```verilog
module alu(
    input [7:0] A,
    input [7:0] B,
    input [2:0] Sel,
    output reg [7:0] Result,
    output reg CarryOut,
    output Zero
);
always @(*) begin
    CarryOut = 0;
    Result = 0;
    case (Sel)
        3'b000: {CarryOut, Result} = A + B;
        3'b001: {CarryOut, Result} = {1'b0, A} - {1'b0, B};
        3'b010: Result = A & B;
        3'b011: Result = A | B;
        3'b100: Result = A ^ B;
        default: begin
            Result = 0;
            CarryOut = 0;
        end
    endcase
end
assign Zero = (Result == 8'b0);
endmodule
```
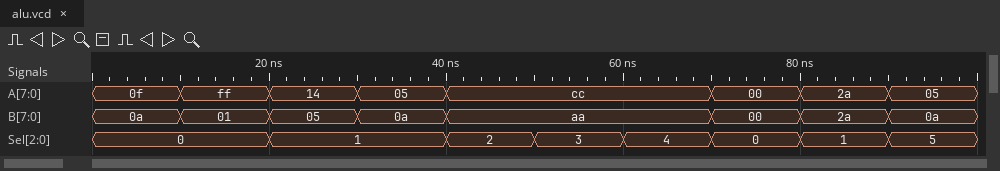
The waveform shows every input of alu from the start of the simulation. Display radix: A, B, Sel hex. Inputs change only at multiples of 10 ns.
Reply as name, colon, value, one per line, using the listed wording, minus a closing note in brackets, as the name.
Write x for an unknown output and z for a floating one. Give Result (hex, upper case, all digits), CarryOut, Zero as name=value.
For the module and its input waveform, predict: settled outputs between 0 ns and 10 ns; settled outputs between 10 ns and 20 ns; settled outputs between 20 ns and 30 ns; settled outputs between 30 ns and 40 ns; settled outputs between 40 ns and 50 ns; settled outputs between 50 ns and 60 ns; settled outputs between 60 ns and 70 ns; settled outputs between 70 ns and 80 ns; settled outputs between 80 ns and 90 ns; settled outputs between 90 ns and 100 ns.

settled outputs between 0 ns and 10 ns: Result=19, CarryOut=0, Zero=0
settled outputs between 10 ns and 20 ns: Result=00, CarryOut=1, Zero=1
settled outputs between 20 ns and 30 ns: Result=0F, CarryOut=0, Zero=0
settled outputs between 30 ns and 40 ns: Result=FB, CarryOut=1, Zero=0
settled outputs between 40 ns and 50 ns: Result=88, CarryOut=0, Zero=0
settled outputs between 50 ns and 60 ns: Result=EE, CarryOut=0, Zero=0
settled outputs between 60 ns and 70 ns: Result=66, CarryOut=0, Zero=0
settled outputs between 70 ns and 80 ns: Result=00, CarryOut=0, Zero=1
settled outputs between 80 ns and 90 ns: Result=00, CarryOut=0, Zero=1
settled outputs between 90 ns and 100 ns: Result=00, CarryOut=0, Zero=1
